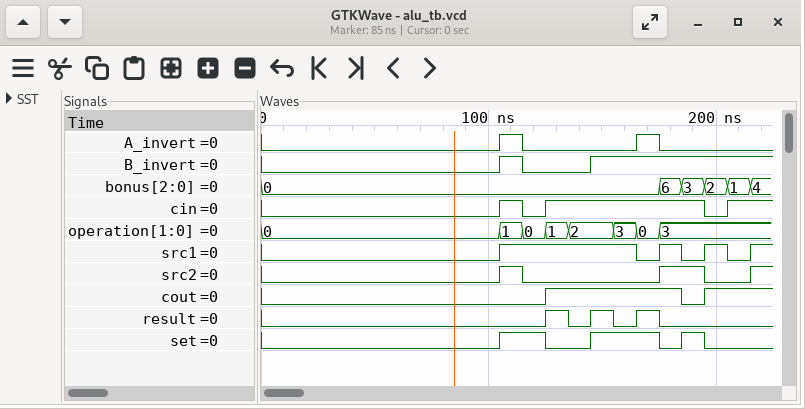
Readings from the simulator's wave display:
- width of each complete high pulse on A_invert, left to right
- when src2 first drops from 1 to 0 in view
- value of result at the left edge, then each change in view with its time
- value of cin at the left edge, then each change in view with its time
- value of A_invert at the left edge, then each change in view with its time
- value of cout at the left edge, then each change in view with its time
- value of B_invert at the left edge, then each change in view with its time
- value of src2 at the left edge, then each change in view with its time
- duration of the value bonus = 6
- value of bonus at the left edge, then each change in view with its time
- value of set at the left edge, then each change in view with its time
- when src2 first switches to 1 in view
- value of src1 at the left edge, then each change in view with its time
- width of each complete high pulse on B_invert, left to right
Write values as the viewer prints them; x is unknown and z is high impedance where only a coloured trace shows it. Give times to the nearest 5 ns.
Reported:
10 ns, 10 ns
115 ns
0, 1 at 125 ns, 0 at 135 ns, 1 at 145 ns, 0 at 155 ns, 1 at 165 ns, 0 at 175 ns
0, 1 at 105 ns, 0 at 115 ns, 1 at 125 ns, 0 at 195 ns, 1 at 205 ns
0, 1 at 105 ns, 0 at 115 ns, 1 at 165 ns, 0 at 175 ns
0, 1 at 125 ns, 0 at 185 ns, 1 at 195 ns
0, 1 at 105 ns, 0 at 115 ns, 1 at 145 ns
0, 1 at 105 ns, 0 at 115 ns, 1 at 175 ns, 0 at 195 ns, 1 at 215 ns
10 ns
0, 6 at 175 ns, 3 at 185 ns, 2 at 195 ns, 1 at 205 ns, 4 at 215 ns
0, 1 at 105 ns, 0 at 125 ns, 1 at 145 ns, 0 at 175 ns, 1 at 185 ns, 0 at 195 ns
105 ns
0, 1 at 105 ns, 0 at 165 ns, 1 at 175 ns, 0 at 185 ns, 1 at 195 ns, 0 at 205 ns, 1 at 215 ns
10 ns
